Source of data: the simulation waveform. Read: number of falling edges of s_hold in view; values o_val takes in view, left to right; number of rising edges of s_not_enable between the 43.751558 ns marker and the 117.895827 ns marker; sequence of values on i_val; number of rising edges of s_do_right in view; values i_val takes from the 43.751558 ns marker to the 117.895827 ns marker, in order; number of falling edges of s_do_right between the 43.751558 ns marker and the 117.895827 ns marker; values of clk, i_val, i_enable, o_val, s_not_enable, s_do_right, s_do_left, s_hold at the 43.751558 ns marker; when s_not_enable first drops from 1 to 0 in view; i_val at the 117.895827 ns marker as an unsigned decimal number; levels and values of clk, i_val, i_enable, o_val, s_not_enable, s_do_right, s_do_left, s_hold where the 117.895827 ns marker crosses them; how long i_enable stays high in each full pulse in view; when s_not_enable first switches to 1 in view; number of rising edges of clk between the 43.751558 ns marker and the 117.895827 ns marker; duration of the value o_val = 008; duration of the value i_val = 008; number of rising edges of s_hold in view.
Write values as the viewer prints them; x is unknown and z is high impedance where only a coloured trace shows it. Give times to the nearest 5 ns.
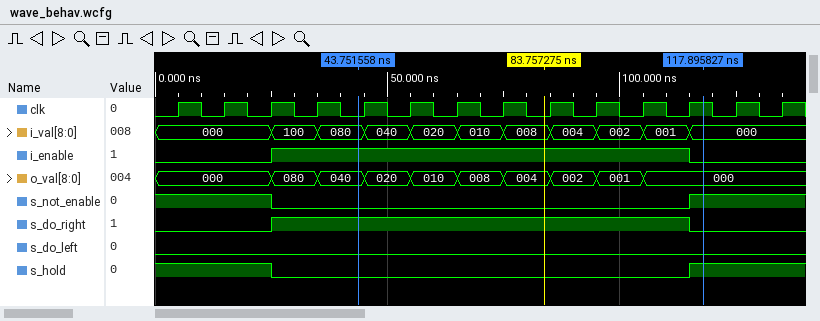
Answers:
1
000, 080, 040, 020, 010, 008, 004, 002, 001, 000
1
000, 100, 080, 040, 020, 010, 008, 004, 002, 001, 000
1
080, 040, 020, 010, 008, 004, 002, 001, 000
1
clk=0, i_val=080, i_enable=1, o_val=040, s_not_enable=0, s_do_right=1, s_do_left=0, s_hold=0
25 ns
0
clk=1, i_val=000, i_enable=0, o_val=000, s_not_enable=1, s_do_right=0, s_do_left=0, s_hold=1
90 ns
115 ns
8
10 ns
10 ns
1
